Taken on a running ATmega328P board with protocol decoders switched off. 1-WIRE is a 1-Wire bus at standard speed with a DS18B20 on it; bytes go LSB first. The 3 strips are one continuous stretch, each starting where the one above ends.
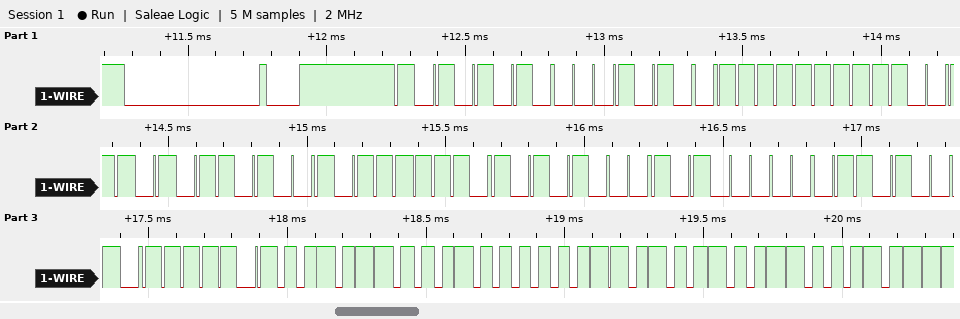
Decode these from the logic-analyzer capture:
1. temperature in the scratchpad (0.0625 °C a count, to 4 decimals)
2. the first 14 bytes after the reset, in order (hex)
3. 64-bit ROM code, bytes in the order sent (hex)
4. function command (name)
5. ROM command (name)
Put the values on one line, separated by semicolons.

35.2500 °C; 55 28 FF B3 96 7E 15 05 96 BE 34 02 4B 46; 28 FF B3 96 7E 15 05 96; Read Scratchpad; Match ROM
